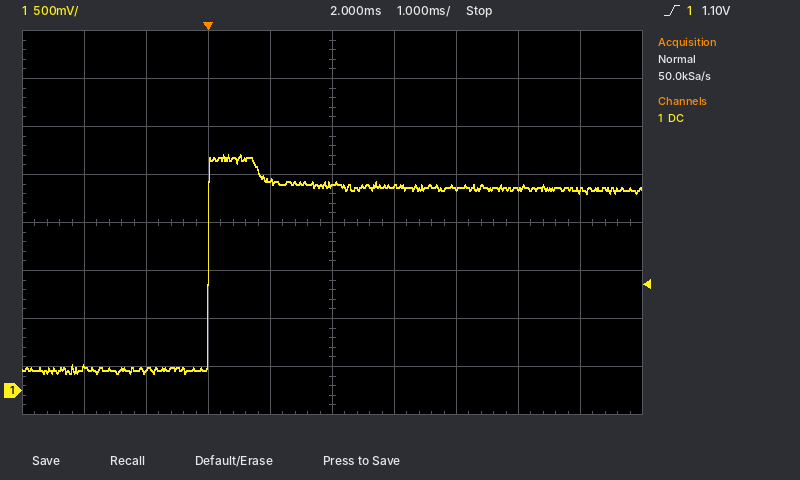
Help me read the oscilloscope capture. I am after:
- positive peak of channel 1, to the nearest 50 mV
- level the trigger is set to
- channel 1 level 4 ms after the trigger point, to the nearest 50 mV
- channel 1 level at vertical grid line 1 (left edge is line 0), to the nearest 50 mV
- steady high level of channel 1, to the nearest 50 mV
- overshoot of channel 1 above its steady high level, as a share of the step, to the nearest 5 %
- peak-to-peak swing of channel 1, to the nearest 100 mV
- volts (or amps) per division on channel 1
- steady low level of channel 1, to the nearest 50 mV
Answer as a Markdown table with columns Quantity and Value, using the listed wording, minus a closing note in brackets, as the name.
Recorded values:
| Quantity | Value |
|---|---|
| positive peak of channel 1, to the nearest 50 mV | 2.45 V |
| level the trigger is set to | 1.10 V |
| channel 1 level 4 ms after the trigger point, to the nearest 50 mV | 2.10 V |
| channel 1 level at vertical grid line 1 (left edge is line 0), to the nearest 50 mV | 250 mV |
| steady high level of channel 1, to the nearest 50 mV | 2.10 V |
| overshoot of channel 1 above its steady high level, as a share of the step, to the nearest 5 % | 20 % |
| peak-to-peak swing of channel 1, to the nearest 100 mV | 2.30 V |
| volts (or amps) per division on channel 1 | 500 mV |
| steady low level of channel 1, to the nearest 50 mV | 200 mV |
